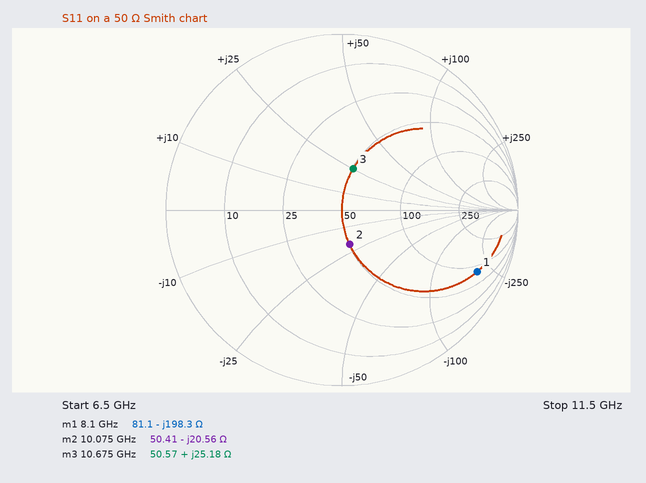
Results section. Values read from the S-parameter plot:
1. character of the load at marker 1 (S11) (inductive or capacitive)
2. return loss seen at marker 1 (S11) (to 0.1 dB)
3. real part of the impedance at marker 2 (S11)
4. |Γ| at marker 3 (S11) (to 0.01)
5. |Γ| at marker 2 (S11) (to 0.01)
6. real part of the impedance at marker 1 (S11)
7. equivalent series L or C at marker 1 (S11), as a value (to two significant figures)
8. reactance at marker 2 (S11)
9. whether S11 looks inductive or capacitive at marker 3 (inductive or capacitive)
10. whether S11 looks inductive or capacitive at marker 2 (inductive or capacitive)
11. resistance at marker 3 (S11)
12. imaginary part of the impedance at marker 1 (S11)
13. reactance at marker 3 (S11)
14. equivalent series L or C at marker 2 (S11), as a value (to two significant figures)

capacitive
1.5 dB
50.41 Ω
0.24
0.20
81.1 Ω
99 fF
-20.56 Ω
inductive
capacitive
50.57 Ω
-198.3 Ω
+25.18 Ω
770 fF
